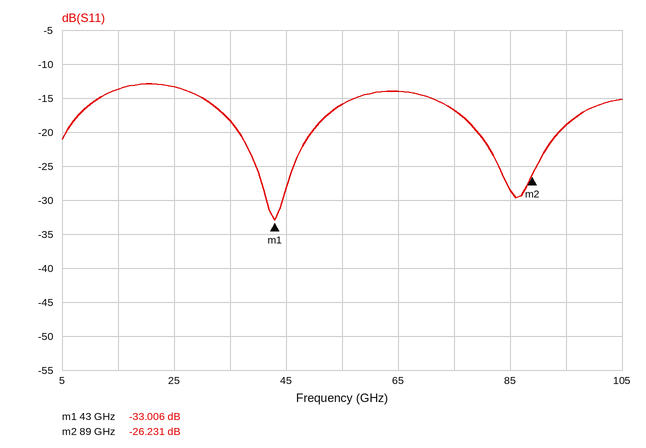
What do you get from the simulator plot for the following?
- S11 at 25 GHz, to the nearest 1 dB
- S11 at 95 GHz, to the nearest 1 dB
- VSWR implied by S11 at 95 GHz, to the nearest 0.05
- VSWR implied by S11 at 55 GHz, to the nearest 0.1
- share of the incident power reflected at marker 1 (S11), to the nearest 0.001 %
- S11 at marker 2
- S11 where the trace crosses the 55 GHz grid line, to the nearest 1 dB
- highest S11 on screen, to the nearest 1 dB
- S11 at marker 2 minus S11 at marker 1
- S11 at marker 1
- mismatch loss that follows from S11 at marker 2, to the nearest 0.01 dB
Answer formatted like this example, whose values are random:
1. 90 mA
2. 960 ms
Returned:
1. -13 dB
2. -19 dB
3. 1.25
4. 1.4
5. 0.050 %
6. -26.231 dB
7. -16 dB
8. -13 dB
9. 6.775 dB
10. -33.006 dB
11. 0.01 dB
